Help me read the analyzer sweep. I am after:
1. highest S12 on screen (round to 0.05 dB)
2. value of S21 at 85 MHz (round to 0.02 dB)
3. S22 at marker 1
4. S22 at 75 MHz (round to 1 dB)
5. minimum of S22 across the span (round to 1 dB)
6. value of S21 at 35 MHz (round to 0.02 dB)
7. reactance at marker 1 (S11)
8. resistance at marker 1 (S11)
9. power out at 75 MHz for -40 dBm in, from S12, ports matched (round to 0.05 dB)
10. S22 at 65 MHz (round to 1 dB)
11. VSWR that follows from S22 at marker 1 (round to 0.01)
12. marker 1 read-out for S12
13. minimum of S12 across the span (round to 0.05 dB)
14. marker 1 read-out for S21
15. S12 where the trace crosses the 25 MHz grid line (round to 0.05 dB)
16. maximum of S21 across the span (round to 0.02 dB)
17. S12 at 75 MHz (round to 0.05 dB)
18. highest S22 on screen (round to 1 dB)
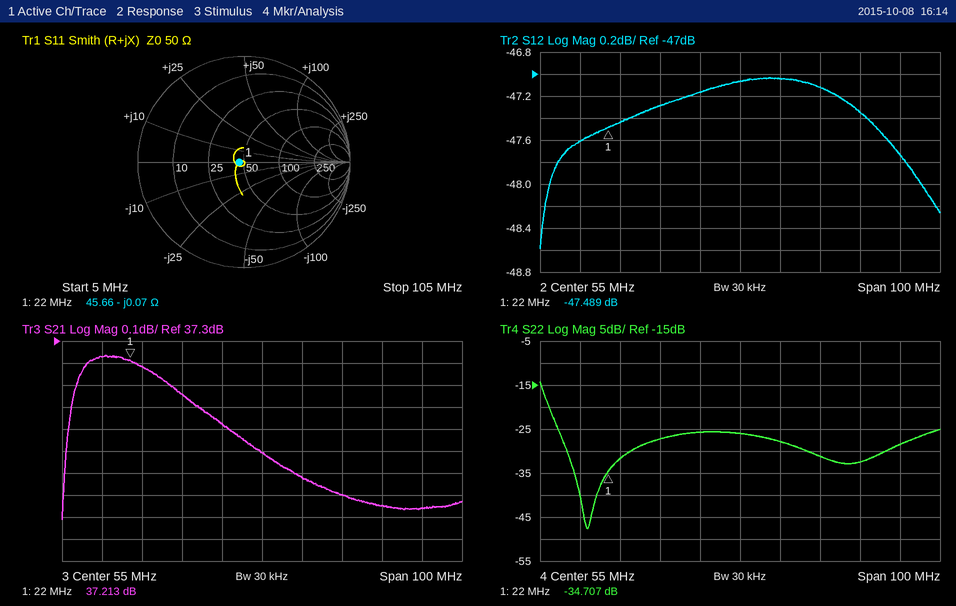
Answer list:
-47.05 dB
36.56 dB
-34.707 dB
-31 dB
-48 dB
37.06 dB
-0.07 Ω
45.66 Ω
-87.10 dBm
-28 dB
1.04
-47.489 dB
-48.60 dB
37.213 dB
-47.45 dB
37.24 dB
-47.10 dB
-14 dB
